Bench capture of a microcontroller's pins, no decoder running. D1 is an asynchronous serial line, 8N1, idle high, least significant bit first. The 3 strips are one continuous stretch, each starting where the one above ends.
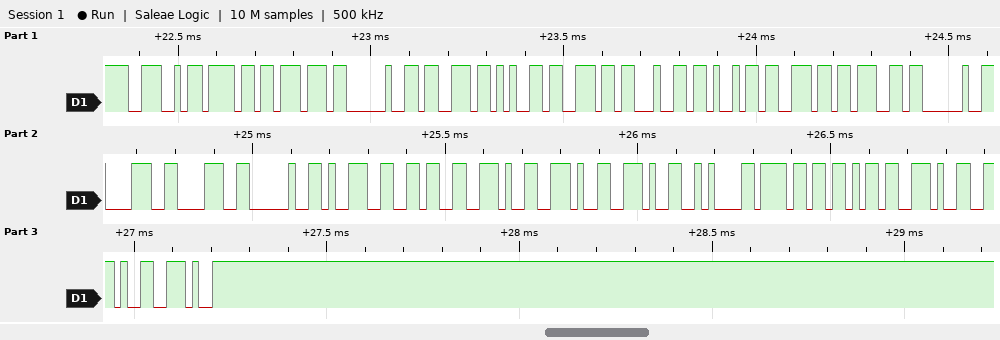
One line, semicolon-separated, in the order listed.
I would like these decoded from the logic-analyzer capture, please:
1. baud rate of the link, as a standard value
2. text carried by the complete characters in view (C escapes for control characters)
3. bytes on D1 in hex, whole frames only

57600 baud; "Now sending 88 96...\nok..."; 4E 6F 77 20 73 65 6E 64 69 6E 67 20 38 38 20 39 36 2E 2E 2E 0A 6F 6B 2E 2E 2E
